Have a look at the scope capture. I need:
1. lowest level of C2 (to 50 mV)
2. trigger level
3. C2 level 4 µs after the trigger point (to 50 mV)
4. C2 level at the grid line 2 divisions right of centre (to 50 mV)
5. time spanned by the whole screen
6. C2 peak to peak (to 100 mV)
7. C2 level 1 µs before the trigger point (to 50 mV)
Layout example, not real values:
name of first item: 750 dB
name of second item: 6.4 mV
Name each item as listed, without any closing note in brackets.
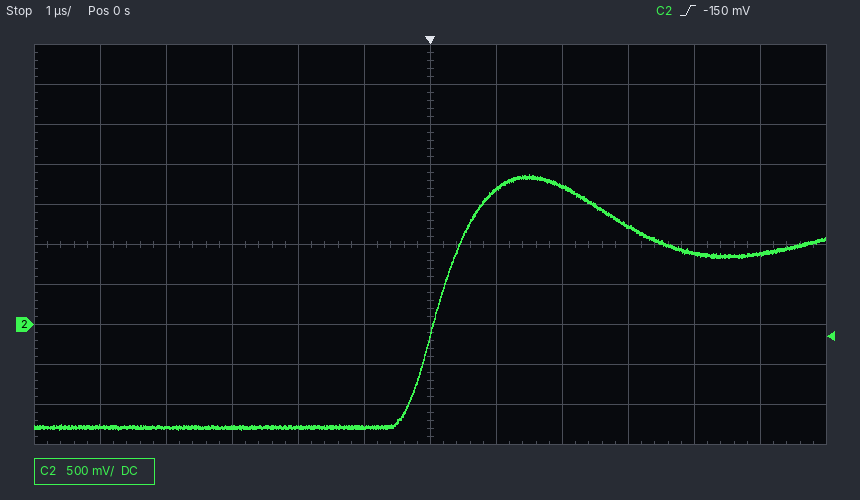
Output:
lowest level of C2: -1.30 V
trigger level: -150 mV
C2 level 4 µs after the trigger point: 900 mV
C2 level at the grid line 2 divisions right of centre: 1.75 V
time spanned by the whole screen: 12 µs
C2 peak to peak: 3.20 V
C2 level 1 µs before the trigger point: -1.30 V
